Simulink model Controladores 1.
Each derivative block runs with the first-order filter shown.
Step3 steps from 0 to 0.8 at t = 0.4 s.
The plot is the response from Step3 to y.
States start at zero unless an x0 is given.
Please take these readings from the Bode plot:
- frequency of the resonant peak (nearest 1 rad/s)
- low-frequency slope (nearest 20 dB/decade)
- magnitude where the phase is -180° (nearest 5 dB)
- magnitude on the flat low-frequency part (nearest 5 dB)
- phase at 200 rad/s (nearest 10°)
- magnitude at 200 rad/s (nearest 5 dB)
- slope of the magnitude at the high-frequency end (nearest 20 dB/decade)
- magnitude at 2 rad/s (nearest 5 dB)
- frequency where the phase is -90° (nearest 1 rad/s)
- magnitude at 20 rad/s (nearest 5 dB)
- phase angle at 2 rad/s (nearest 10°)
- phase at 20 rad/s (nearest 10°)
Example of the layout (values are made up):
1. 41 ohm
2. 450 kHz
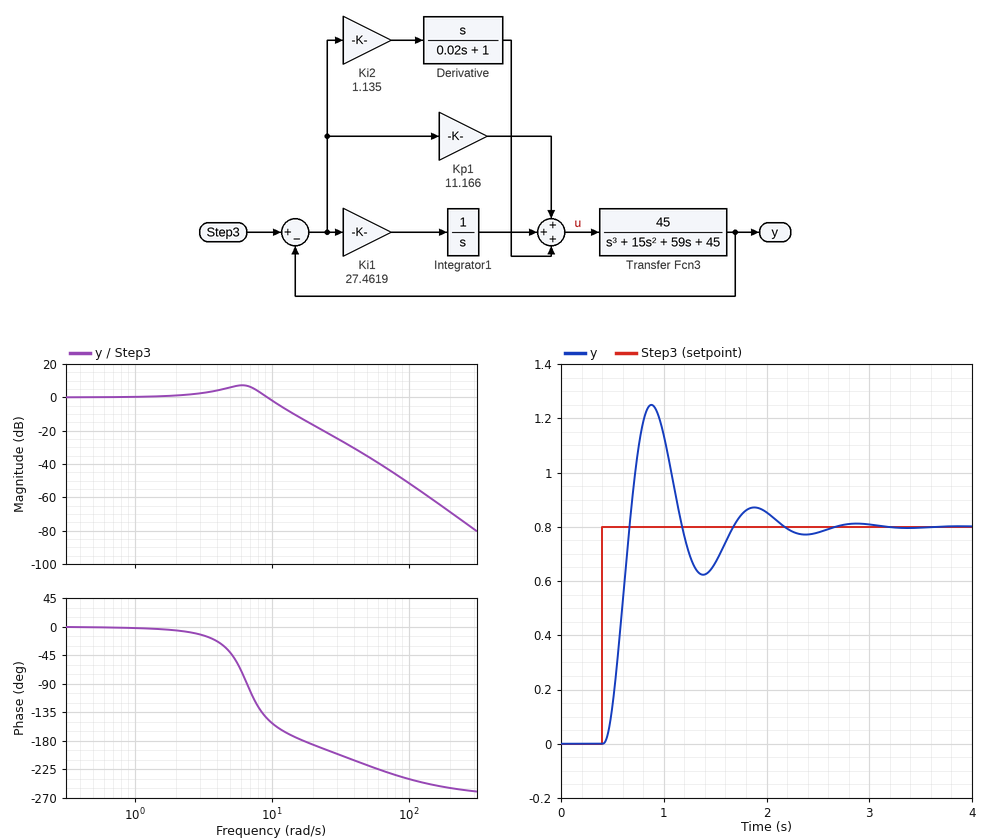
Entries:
1. 6 rad/s
2. 0 dB/decade
3. -15 dB
4. 0 dB
5. -250°
6. -70 dB
7. -60 dB/decade
8. 0 dB
9. 7 rad/s
10. -15 dB
11. -10°
12. -190°
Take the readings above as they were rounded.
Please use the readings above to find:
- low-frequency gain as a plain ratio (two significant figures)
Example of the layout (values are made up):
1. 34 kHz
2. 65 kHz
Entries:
1. 1.0
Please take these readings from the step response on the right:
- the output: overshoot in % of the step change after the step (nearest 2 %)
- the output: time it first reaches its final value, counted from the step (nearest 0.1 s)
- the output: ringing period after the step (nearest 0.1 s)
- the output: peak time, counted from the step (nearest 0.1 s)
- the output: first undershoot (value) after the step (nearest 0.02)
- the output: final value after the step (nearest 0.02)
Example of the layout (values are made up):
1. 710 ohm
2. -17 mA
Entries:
1. 56 %
2. 0.3 s
3. 1.0 s
4. 0.5 s
5. 0.62
6. 0.80
